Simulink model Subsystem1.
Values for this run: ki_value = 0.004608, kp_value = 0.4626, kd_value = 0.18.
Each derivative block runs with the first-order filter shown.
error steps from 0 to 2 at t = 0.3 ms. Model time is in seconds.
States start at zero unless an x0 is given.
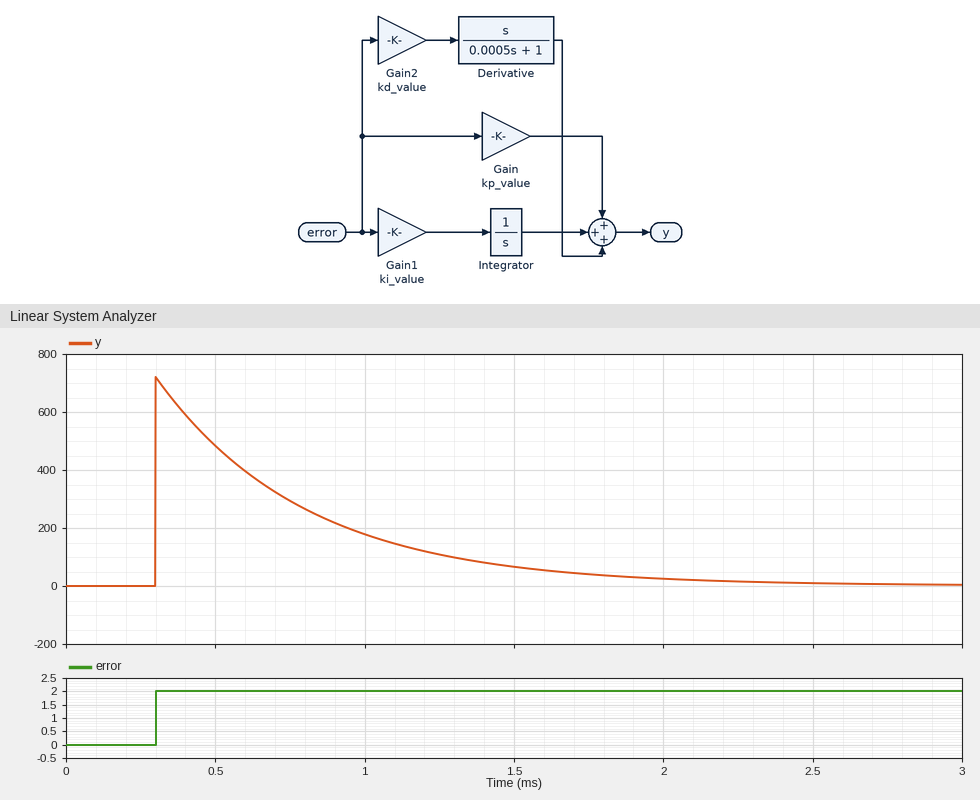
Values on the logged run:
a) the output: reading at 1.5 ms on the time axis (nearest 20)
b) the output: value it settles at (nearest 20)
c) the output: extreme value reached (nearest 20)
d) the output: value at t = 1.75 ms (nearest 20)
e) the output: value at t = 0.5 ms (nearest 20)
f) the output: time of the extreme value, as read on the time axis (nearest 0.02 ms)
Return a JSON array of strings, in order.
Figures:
["60", "0", "720", "40", "480", "0.30 ms"]
